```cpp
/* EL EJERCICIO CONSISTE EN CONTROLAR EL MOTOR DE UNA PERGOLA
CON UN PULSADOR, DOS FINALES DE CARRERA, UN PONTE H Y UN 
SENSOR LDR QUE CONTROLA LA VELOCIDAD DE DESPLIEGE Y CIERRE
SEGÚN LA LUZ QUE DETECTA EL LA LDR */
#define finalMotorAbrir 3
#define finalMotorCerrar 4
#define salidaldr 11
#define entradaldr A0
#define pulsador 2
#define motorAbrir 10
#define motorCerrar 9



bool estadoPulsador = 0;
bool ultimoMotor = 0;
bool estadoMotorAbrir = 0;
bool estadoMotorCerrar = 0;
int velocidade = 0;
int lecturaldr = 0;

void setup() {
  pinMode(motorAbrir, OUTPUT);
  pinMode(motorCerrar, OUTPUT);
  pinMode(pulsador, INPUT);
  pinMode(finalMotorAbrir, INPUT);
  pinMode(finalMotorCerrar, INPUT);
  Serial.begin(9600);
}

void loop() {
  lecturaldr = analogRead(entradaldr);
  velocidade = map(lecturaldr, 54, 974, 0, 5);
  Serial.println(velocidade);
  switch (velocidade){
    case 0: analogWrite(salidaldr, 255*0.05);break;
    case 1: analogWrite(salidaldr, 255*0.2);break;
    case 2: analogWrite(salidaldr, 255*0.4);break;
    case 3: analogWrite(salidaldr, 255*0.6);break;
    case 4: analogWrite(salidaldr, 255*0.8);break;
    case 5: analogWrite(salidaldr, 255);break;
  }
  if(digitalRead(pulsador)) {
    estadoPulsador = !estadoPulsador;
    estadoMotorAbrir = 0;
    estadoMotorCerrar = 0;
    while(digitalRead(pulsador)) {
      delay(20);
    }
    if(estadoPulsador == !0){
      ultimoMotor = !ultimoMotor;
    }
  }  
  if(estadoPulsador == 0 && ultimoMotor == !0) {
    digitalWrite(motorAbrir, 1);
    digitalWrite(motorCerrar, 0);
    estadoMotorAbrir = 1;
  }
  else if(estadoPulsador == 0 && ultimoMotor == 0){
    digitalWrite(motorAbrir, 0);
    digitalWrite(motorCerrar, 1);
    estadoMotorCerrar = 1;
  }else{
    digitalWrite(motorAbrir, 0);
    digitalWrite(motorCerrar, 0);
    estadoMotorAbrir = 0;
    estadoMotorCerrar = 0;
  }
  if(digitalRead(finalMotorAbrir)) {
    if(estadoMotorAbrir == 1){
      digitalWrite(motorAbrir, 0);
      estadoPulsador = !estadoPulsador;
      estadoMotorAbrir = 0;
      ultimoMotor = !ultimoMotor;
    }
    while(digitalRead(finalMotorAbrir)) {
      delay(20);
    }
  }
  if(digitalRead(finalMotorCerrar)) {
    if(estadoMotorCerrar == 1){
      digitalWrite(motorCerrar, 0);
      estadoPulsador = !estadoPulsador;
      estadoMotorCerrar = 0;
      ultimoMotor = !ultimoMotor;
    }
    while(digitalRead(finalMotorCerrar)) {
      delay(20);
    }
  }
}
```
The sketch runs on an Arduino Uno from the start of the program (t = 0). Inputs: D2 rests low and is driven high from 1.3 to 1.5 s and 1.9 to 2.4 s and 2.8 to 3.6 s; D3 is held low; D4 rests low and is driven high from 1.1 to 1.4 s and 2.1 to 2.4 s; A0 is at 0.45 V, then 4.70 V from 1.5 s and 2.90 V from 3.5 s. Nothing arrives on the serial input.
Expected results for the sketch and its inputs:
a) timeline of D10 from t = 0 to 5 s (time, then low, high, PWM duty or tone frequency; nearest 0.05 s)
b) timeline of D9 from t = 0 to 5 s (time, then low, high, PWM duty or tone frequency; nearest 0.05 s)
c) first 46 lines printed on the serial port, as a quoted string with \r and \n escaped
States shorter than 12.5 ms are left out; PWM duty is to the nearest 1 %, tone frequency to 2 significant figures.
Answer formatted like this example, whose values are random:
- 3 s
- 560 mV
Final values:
- 0 s low; 1.5 s high; 2.4 s low
- 0 s high; 1.1 s low; 3.6 s high
- "0\r\n0\r\n0\r\n0\r\n0\r\n0\r\n0\r\n0\r\n0\r\n0\r\n0\r\n0\r\n0\r\n0\r\n0\r\n0\r\n0\r\n0\r\n0\r\n0\r\n0\r\n0\r\n0\r\n0\r\n0\r\n0\r\n0\r\n0\r\n0\r\n0\r\n0\r\n0\r\n0\r\n0\r\n0\r\n0\r\n0\r\n0\r\n0\r\n0\r\n0\r\n0\r\n0\r\n0\r\n0\r\n0\r\n"
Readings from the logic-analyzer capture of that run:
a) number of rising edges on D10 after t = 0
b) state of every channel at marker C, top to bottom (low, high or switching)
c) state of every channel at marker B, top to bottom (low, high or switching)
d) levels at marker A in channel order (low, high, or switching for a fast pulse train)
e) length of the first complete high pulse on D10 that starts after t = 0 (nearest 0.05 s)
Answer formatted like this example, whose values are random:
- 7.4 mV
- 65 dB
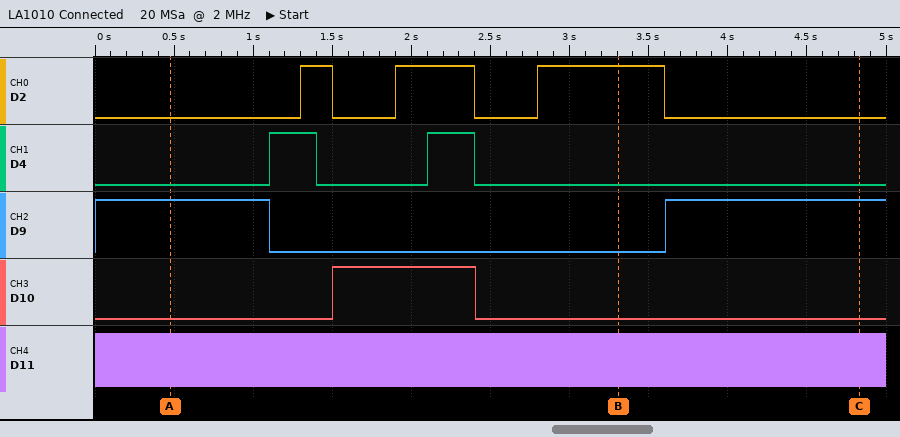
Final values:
- 1
- D2 low, D4 low, D9 high, D10 low, D11 switching
- D2 high, D4 low, D9 low, D10 low, D11 switching
- D2 low, D4 low, D9 high, D10 low, D11 switching
- 0.90 s
